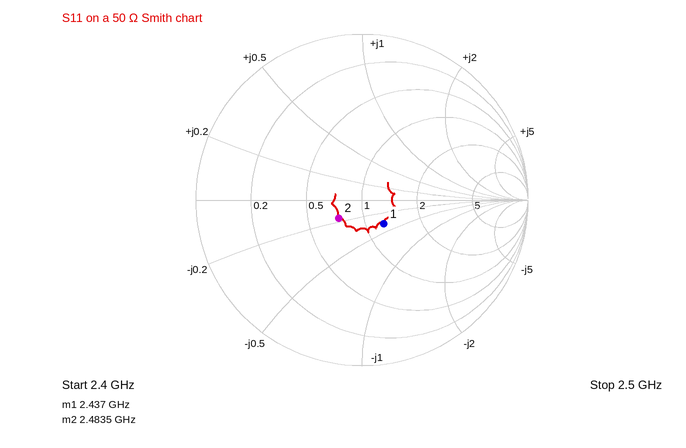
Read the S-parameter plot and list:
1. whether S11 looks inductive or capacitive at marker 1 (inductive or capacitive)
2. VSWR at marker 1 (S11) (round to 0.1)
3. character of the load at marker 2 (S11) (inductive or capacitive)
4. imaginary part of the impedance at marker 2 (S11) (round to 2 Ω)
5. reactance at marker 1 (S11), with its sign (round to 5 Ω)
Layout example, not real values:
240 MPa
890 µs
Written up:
capacitive
1.5
capacitive
-8 Ω
-20 Ω
